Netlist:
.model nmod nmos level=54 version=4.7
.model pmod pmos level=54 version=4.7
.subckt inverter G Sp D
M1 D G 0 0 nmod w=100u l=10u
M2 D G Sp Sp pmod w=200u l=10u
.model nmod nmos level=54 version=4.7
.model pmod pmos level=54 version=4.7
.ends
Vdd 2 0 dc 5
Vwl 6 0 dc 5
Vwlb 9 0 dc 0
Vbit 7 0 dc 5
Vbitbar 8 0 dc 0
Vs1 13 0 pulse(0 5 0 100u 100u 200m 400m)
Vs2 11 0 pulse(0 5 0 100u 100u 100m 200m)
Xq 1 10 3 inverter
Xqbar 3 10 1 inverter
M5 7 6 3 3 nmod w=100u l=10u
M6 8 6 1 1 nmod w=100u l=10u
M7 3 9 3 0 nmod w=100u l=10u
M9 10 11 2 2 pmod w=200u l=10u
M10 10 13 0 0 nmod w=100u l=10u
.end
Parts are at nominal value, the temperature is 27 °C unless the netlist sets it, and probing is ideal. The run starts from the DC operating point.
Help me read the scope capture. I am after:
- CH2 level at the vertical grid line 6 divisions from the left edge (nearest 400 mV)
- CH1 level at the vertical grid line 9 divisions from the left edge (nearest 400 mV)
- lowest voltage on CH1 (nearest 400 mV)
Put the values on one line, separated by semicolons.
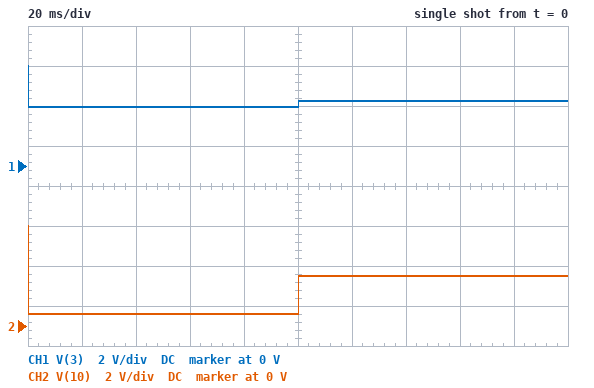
2.4 V; 3.2 V; 2.8 V
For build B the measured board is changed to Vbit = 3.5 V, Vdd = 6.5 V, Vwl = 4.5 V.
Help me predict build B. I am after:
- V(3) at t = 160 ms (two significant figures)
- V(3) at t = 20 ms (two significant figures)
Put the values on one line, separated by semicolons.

3.3 V; 2.5 V
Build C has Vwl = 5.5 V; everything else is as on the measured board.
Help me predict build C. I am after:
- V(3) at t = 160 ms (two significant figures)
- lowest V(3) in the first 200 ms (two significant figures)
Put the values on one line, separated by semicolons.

3.5 V; 3.2 V
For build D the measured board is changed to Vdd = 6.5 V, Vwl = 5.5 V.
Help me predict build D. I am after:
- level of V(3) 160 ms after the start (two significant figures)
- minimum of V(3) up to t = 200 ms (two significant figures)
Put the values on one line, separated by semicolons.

4.0 V; 3.2 V
